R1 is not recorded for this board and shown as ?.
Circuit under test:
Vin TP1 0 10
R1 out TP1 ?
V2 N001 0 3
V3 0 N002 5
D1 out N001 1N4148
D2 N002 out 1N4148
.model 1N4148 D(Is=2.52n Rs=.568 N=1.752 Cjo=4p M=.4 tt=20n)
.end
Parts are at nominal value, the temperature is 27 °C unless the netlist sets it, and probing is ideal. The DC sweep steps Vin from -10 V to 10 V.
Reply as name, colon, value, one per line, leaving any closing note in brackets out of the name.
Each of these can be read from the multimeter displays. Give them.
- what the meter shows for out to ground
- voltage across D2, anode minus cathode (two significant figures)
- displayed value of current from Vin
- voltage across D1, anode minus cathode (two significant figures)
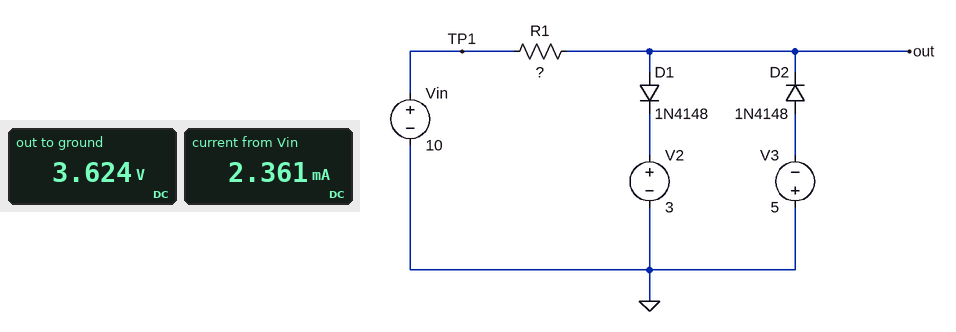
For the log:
what the meter shows for out to ground: 3.624 V
voltage across D2, anode minus cathode: -8.6 V
displayed value of current from Vin: 2.361 mA
voltage across D1, anode minus cathode: 620 mV
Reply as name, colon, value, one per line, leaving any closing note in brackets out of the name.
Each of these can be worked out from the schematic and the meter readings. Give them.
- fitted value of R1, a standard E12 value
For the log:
fitted value of R1, a standard E12 value: 2.7 kΩ
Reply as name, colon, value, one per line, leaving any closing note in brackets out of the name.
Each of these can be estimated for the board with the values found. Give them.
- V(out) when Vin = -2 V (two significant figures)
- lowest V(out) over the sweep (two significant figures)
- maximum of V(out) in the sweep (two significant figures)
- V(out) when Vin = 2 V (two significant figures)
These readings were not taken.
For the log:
V(out) when Vin = -2 V: -2.0 V
lowest V(out) over the sweep: -5.6 V
maximum of V(out) in the sweep: 3.6 V
V(out) when Vin = 2 V: 2.0 V
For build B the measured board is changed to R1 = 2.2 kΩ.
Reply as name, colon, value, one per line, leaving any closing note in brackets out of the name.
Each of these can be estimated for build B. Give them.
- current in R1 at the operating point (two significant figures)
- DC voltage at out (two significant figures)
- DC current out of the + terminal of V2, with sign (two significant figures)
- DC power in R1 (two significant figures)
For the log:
current in R1 at the operating point: 2.9 mA
DC voltage at out: 3.6 V
DC current out of the + terminal of V2, with sign: -2.9 mA
DC power in R1: 18 mW
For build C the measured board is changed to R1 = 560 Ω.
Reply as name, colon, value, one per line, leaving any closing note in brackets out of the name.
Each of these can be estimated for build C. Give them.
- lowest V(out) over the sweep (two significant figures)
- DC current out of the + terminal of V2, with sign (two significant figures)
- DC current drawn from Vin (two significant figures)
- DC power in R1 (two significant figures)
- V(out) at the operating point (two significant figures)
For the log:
lowest V(out) over the sweep: -5.7 V
DC current out of the + terminal of V2, with sign: -11 mA
DC current drawn from Vin: 11 mA
DC power in R1: 71 mW
V(out) at the operating point: 3.7 V
